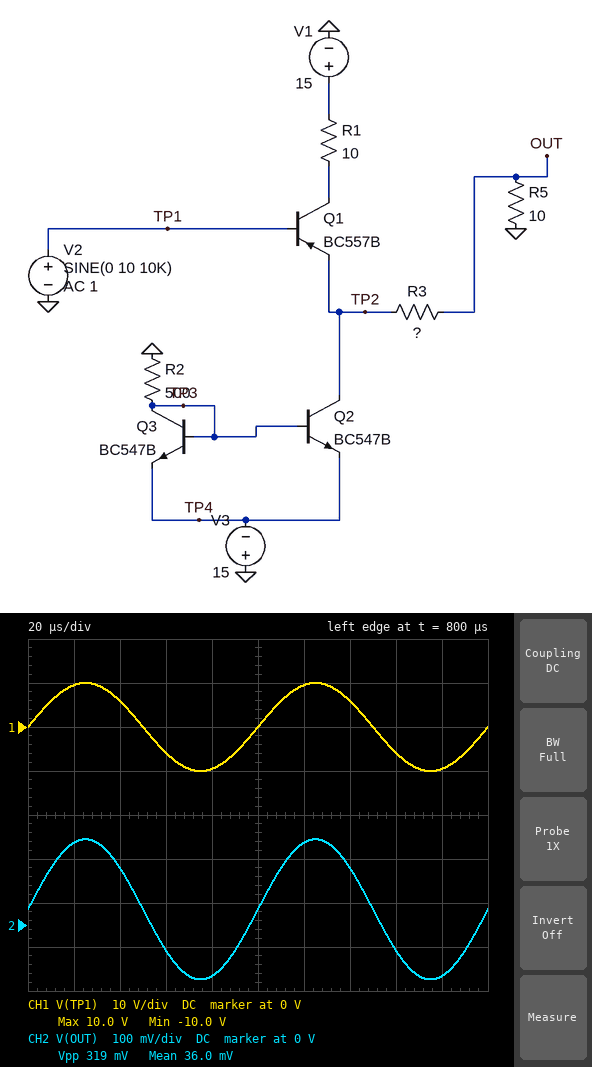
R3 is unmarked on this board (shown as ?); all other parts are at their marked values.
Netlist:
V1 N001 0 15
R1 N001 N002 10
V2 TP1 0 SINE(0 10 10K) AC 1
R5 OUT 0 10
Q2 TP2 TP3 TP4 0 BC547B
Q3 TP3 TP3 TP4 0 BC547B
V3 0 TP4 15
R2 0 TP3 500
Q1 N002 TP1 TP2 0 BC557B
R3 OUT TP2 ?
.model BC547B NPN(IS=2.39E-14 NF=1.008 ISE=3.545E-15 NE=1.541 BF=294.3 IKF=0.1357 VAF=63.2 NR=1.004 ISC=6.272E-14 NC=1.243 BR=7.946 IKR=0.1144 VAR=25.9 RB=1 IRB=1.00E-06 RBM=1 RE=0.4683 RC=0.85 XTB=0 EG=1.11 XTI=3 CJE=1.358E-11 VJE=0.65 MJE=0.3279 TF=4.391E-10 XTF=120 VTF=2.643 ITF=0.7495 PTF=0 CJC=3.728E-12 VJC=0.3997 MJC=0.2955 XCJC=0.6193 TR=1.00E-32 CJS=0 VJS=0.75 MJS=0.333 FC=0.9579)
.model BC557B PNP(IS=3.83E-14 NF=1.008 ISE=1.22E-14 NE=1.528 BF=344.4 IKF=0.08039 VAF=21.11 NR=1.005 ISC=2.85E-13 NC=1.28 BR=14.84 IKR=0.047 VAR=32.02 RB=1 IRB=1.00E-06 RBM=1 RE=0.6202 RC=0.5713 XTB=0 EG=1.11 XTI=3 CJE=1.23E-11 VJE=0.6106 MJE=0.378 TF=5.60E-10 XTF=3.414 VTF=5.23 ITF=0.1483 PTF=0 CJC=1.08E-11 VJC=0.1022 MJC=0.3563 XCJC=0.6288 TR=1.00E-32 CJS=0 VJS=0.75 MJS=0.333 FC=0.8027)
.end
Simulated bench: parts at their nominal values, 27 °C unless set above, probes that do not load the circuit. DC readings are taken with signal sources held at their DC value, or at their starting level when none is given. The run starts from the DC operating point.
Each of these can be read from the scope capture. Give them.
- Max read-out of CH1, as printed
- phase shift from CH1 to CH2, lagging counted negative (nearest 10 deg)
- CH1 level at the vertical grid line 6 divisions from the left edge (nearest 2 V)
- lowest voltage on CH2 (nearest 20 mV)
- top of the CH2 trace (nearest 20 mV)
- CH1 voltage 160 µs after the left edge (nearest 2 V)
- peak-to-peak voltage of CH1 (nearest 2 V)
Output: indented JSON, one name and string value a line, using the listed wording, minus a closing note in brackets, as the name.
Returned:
{
  "Max read-out of CH1, as printed": "10.0 V",
  "phase shift from CH1 to CH2, lagging counted negative": "0 deg",
  "CH1 level at the vertical grid line 6 divisions from the left edge": "10 V",
  "lowest voltage on CH2": "-120 mV",
  "top of the CH2 trace": "200 mV",
  "CH1 voltage 160 µs after the left edge": "-6 V",
  "peak-to-peak voltage of CH1": "20 V"
}
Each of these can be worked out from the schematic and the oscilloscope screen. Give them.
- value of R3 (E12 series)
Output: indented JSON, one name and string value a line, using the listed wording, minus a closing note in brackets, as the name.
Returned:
{
  "value of R3": "560 Ω"
}
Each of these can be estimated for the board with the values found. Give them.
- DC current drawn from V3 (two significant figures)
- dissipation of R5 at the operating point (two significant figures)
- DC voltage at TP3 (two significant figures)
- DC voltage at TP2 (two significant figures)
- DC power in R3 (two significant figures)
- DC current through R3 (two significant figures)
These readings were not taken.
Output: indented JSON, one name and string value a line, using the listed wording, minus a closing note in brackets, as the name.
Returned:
{
  "DC current drawn from V3": "62 mA",
  "dissipation of R5 at the operating point": "130 µW",
  "DC voltage at TP3": "-14 V",
  "DC voltage at TP2": "2.0 V",
  "DC power in R3": "7.2 mW",
  "DC current through R3": "3.6 mA"
}
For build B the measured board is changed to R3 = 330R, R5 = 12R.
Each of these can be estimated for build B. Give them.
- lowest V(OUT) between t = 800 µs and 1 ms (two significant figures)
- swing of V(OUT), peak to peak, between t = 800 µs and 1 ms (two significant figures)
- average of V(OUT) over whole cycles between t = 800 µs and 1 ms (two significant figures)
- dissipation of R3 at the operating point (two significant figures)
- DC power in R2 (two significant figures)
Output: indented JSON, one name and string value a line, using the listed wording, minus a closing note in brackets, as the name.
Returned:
{
  "lowest V(OUT) between t = 800 µs and 1 ms": "-250 mV",
  "swing of V(OUT), peak to peak, between t = 800 µs and 1 ms": "640 mV",
  "average of V(OUT) over whole cycles between t = 800 µs and 1 ms": "71 mV",
  "dissipation of R3 at the operating point": "12 mW",
  "DC power in R2": "410 mW"
}
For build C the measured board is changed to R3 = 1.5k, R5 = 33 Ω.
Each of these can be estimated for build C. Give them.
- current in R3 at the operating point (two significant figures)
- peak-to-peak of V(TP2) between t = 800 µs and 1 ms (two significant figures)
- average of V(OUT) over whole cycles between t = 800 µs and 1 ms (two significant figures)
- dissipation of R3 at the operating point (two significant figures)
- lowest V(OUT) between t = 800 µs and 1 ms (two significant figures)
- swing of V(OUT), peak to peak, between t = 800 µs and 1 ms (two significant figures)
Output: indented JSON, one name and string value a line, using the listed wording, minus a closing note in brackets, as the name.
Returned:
{
  "current in R3 at the operating point": "1.3 mA",
  "peak-to-peak of V(TP2) between t = 800 µs and 1 ms": "18 V",
  "average of V(OUT) over whole cycles between t = 800 µs and 1 ms": "44 mV",
  "dissipation of R3 at the operating point": "2.7 mW",
  "lowest V(OUT) between t = 800 µs and 1 ms": "-150 mV",
  "swing of V(OUT), peak to peak, between t = 800 µs and 1 ms": "390 mV"
}
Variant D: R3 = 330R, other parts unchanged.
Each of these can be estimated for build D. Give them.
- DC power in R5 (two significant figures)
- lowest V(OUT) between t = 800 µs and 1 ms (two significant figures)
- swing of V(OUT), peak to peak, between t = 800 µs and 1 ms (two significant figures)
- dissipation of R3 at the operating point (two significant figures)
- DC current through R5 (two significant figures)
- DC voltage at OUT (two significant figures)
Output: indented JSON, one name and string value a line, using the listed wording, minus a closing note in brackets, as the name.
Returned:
{
  "DC power in R5": "360 µW",
  "lowest V(OUT) between t = 800 µs and 1 ms": "-210 mV",
  "swing of V(OUT), peak to peak, between t = 800 µs and 1 ms": "530 mV",
  "dissipation of R3 at the operating point": "12 mW",
  "DC current through R5": "6.0 mA",
  "DC voltage at OUT": "60 mV"
}
